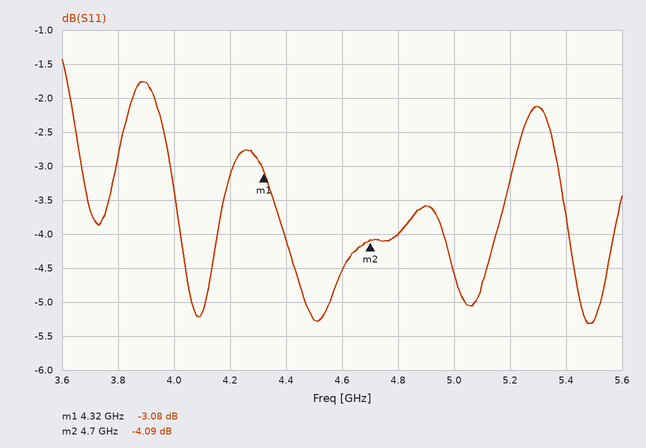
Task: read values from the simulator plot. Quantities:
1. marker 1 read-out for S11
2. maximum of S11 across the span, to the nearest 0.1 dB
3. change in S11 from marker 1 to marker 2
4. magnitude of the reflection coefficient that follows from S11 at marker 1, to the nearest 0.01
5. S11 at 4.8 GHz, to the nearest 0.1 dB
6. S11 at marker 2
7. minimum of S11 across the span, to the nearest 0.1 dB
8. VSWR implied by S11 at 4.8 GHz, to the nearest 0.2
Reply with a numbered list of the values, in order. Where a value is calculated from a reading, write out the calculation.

1. -3.08 dB
2. -1.4 dB
3. -4.09 − (-3.08) = -1.01 dB
4. 10^(-3.08/20) ≈ 0.70
5. -4.0 dB
6. -4.09 dB
7. -5.3 dB
8. |Γ| = 10^(-4/20) = 0.6310; VSWR = (1 + 0.6310)/(1 − 0.6310) ≈ 4.4
